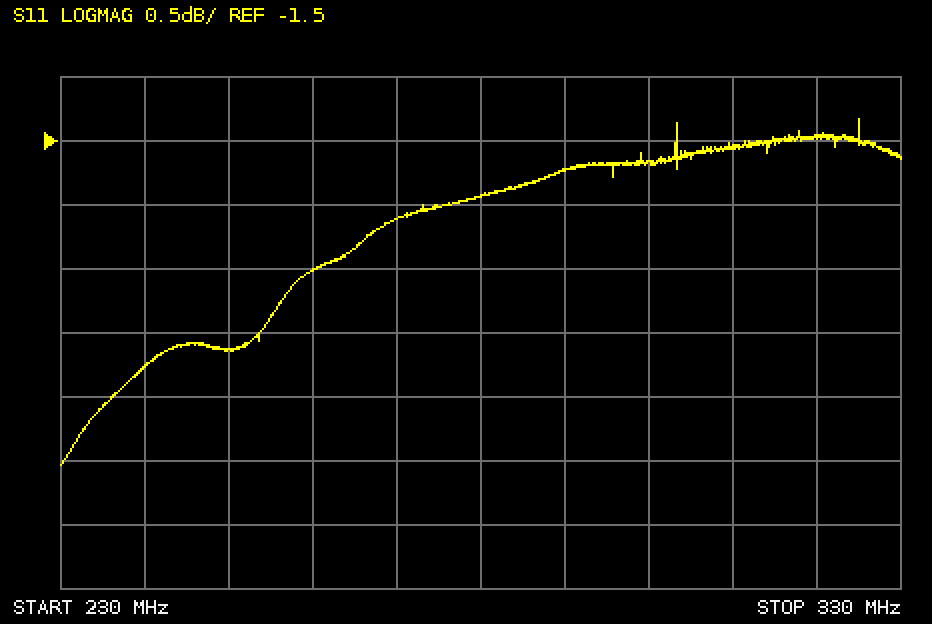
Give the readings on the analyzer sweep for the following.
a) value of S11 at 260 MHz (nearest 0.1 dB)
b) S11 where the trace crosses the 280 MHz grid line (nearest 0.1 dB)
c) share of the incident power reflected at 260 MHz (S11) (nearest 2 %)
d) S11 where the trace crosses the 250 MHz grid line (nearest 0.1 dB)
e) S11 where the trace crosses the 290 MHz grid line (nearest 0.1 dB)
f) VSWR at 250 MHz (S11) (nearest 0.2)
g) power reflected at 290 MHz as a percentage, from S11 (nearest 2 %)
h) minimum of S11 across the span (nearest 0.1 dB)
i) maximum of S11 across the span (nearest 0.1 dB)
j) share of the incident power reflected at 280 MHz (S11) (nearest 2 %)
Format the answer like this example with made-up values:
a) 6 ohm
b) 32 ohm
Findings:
a) -2.5 dB
b) -1.9 dB
c) 56 %
d) -3.1 dB
e) -1.7 dB
f) 5.6
g) 68 %
h) -4.0 dB
i) -1.3 dB
j) 64 %
